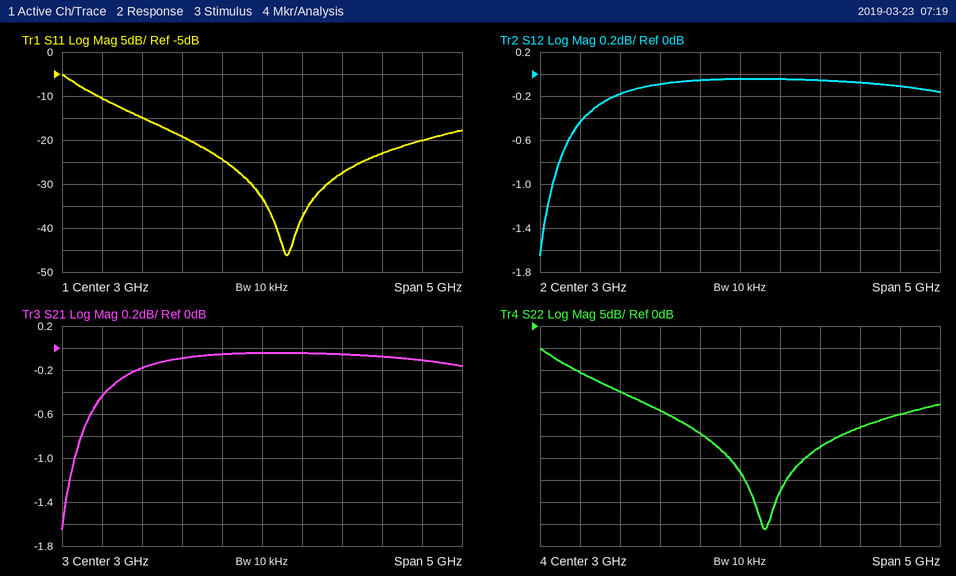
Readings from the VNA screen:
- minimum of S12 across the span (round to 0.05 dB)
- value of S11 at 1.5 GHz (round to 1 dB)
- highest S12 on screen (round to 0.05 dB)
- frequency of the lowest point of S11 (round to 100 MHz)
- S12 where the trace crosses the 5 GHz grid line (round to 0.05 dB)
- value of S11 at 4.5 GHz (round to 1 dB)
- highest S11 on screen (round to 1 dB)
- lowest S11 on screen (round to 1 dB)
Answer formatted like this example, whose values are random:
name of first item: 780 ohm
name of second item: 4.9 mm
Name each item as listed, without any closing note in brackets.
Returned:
minimum of S12 across the span: -1.65 dB
value of S11 at 1.5 GHz: -15 dB
highest S12 on screen: -0.05 dB
frequency of the lowest point of S11: 3.3 GHz
S12 where the trace crosses the 5 GHz grid line: -0.10 dB
value of S11 at 4.5 GHz: -23 dB
highest S11 on screen: -5 dB
lowest S11 on screen: -46 dB
